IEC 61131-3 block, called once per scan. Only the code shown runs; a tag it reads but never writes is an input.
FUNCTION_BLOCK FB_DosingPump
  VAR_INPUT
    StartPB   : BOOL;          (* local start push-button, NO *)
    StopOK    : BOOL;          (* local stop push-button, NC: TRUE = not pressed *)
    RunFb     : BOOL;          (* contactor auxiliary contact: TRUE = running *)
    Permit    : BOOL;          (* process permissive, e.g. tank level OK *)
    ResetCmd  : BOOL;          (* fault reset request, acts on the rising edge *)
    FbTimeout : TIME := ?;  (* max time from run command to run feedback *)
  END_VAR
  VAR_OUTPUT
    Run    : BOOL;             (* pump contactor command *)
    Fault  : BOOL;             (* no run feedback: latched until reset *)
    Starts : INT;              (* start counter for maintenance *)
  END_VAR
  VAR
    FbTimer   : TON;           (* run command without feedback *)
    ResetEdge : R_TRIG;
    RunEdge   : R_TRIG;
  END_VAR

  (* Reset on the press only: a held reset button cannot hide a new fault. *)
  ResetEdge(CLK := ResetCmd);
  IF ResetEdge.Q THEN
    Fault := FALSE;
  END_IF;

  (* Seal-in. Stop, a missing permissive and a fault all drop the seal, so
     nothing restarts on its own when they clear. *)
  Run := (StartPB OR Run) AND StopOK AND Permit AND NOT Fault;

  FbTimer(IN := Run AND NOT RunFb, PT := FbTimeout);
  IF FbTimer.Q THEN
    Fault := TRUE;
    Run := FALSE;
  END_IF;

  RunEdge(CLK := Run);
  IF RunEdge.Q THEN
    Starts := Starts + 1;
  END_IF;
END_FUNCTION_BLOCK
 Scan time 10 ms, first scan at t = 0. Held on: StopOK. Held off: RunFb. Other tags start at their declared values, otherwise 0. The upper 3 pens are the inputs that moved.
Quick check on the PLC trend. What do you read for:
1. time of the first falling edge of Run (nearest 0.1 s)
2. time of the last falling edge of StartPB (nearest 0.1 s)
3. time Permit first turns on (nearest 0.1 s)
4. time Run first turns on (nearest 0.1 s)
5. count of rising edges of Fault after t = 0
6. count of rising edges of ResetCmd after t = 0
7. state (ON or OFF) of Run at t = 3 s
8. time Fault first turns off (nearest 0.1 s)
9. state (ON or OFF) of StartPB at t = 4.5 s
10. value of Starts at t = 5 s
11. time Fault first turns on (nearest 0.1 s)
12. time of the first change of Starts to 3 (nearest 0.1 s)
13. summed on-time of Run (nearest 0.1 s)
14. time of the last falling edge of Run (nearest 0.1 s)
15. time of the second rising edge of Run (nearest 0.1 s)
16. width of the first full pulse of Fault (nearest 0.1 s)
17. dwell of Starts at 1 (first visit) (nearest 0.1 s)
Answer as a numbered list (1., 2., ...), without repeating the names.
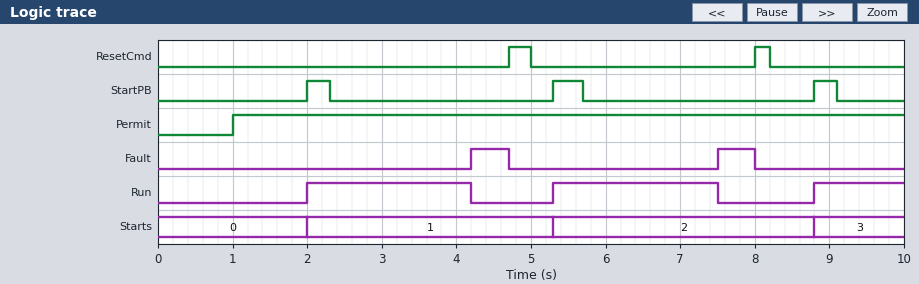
1. 4.2 s
2. 9.1 s
3. 1.0 s
4. 2.0 s
5. 2
6. 2
7. ON
8. 4.7 s
9. OFF
10. 1
11. 4.2 s
12. 8.8 s
13. 5.6 s
14. 7.5 s
15. 5.3 s
16. 0.5 s
17. 3.3 s
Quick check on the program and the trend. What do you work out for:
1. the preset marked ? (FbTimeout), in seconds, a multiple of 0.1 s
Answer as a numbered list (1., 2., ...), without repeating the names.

1. 2.2 s
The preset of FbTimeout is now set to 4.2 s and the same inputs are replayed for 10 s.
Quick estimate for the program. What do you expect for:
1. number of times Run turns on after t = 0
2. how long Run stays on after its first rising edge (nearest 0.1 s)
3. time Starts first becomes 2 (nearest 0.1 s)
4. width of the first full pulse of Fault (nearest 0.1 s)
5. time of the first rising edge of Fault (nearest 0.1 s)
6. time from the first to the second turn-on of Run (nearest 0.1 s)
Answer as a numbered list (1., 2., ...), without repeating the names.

1. 2
2. 4.2 s
3. 8.8 s
4. 1.8 s
5. 6.2 s
6. 6.8 s
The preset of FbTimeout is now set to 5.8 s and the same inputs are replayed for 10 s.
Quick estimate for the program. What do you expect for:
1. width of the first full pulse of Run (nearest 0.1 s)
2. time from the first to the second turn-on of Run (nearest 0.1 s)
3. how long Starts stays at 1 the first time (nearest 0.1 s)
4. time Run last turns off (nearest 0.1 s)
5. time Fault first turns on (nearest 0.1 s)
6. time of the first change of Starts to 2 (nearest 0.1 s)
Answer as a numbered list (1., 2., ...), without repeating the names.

1. 5.8 s
2. 6.8 s
3. 6.8 s
4. 7.8 s
5. 7.8 s
6. 8.8 s
